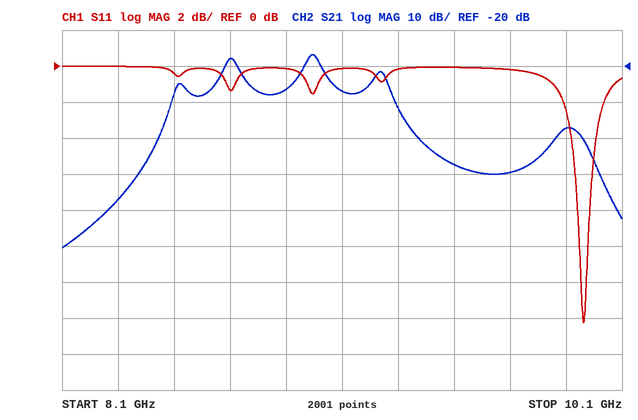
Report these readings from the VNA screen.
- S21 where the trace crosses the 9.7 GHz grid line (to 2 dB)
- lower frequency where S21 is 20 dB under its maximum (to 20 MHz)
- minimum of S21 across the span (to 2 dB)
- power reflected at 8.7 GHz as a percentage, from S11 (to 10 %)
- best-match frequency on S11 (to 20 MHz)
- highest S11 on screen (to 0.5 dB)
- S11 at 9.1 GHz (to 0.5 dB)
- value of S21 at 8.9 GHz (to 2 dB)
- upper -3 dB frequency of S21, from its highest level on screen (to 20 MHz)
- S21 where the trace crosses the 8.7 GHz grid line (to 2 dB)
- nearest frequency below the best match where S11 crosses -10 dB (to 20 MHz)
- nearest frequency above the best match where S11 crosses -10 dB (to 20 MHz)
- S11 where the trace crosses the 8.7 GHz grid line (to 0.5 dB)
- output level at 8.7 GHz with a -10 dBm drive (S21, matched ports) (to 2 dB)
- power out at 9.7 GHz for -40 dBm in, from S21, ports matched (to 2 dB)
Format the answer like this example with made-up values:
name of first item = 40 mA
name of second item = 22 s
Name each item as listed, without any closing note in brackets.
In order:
S21 where the trace crosses the 9.7 GHz grid line = -50 dB
lower frequency where S21 is 20 dB under its maximum = 8.46 GHz
minimum of S21 across the span = -70 dB
power reflected at 8.7 GHz as a percentage, from S11 = 70 %
best-match frequency on S11 = 9.96 GHz
highest S11 on screen = 0.0 dB
S11 at 9.1 GHz = 0.0 dB
value of S21 at 8.9 GHz = -26 dB
upper -3 dB frequency of S21, from its highest level on screen = 9.02 GHz
S21 where the trace crosses the 8.7 GHz grid line = -18 dB
nearest frequency below the best match where S11 crosses -10 dB = 9.94 GHz
nearest frequency above the best match where S11 crosses -10 dB = 9.98 GHz
S11 where the trace crosses the 8.7 GHz grid line = -1.5 dB
output level at 8.7 GHz with a -10 dBm drive (S21, matched ports) = -28 dBm
power out at 9.7 GHz for -40 dBm in, from S21, ports matched = -90 dBm
